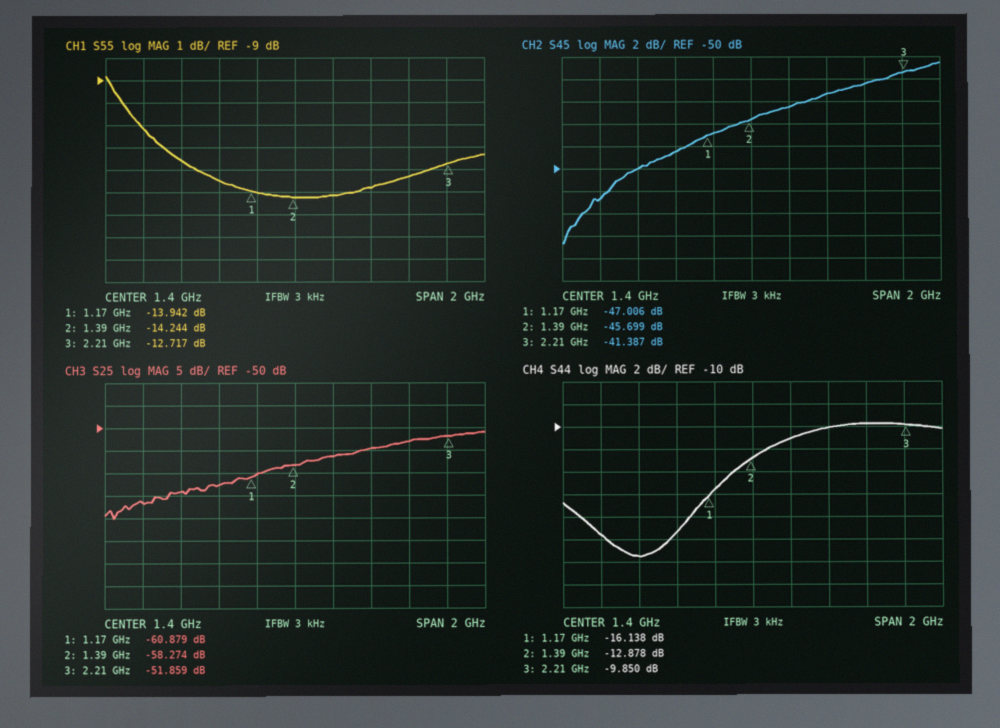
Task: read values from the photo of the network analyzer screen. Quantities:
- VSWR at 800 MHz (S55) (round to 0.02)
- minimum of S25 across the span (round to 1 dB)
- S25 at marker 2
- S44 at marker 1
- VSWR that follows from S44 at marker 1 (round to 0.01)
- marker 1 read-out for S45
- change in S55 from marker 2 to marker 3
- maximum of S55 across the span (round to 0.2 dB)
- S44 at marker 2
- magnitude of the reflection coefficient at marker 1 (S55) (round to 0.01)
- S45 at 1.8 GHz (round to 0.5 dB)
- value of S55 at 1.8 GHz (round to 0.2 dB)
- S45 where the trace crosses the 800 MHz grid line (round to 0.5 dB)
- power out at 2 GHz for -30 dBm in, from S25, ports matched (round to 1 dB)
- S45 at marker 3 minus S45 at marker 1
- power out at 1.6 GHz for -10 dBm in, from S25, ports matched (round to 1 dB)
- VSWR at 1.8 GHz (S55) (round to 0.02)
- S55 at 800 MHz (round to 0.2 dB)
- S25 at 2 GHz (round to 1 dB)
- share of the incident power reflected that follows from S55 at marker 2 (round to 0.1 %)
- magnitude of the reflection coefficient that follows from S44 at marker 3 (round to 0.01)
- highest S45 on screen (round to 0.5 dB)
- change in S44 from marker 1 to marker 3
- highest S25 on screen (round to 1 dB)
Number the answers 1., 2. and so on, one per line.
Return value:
1. 1.62
2. -70 dB
3. -58.274 dB
4. -16.138 dB
5. 1.37
6. -47.006 dB
7. 1.527 dB
8. -8.8 dB
9. -12.878 dB
10. 0.20
11. -43.5 dB
12. -13.8 dB
13. -50.0 dB
14. -83 dBm
15. 5.619 dB
16. -66 dBm
17. 1.52
18. -12.6 dB
19. -53 dB
20. 3.8 %
21. 0.32
22. -40.5 dB
23. 6.288 dB
24. -51 dB
